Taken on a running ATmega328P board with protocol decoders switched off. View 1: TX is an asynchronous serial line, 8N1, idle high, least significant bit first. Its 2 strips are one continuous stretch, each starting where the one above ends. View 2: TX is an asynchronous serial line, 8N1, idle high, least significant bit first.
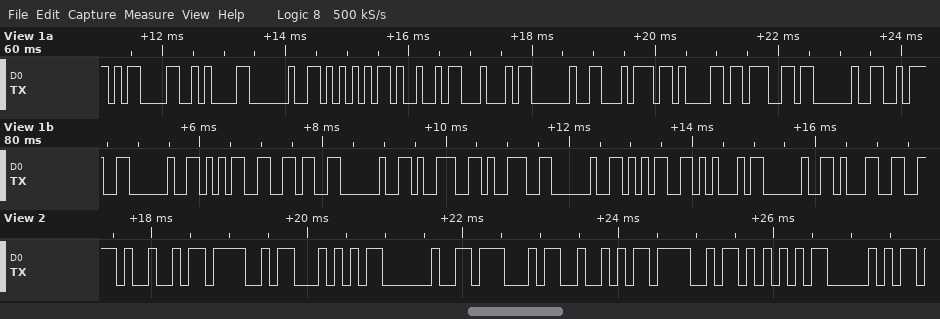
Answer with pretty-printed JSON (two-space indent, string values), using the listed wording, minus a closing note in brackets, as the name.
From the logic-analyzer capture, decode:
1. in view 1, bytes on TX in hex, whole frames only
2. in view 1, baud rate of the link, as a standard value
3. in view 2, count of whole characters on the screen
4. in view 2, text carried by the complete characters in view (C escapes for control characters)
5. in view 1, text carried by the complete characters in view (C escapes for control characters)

{
  "in view 1, bytes on TX in hex, whole frames only": "0x0D 0x0A 0x20 0x55 0x49 0x44 0x20 0x74 0x61 0x67 0x20 0x3A 0x20 0x35 0x36 0x20 0x39 0x39 0x20 0x35 0x45 0x20 0x31",
  "in view 1, baud rate of the link, as a standard value": "9600 baud",
  "in view 2, count of whole characters on the screen": "9",
  "in view 2, text carried by the complete characters in view": "\"IOT GROUP\"",
  "in view 1, text carried by the complete characters in view": "\"\\r\\n UID tag : 56 99 5E 1\""
}
